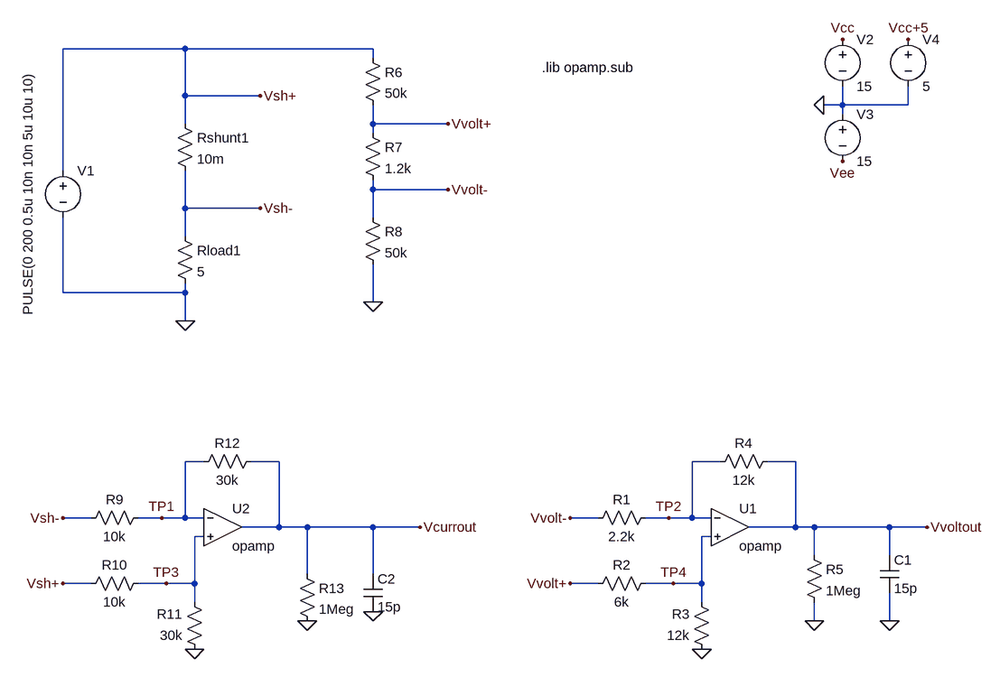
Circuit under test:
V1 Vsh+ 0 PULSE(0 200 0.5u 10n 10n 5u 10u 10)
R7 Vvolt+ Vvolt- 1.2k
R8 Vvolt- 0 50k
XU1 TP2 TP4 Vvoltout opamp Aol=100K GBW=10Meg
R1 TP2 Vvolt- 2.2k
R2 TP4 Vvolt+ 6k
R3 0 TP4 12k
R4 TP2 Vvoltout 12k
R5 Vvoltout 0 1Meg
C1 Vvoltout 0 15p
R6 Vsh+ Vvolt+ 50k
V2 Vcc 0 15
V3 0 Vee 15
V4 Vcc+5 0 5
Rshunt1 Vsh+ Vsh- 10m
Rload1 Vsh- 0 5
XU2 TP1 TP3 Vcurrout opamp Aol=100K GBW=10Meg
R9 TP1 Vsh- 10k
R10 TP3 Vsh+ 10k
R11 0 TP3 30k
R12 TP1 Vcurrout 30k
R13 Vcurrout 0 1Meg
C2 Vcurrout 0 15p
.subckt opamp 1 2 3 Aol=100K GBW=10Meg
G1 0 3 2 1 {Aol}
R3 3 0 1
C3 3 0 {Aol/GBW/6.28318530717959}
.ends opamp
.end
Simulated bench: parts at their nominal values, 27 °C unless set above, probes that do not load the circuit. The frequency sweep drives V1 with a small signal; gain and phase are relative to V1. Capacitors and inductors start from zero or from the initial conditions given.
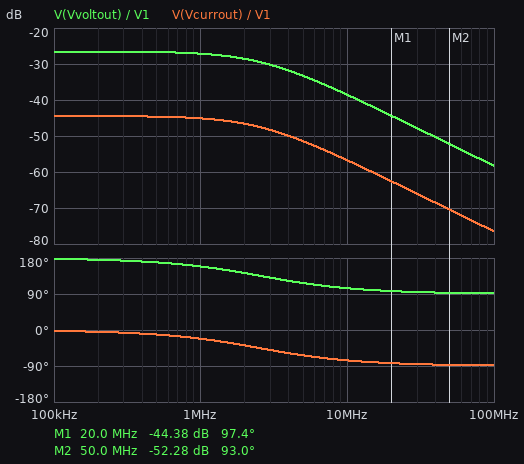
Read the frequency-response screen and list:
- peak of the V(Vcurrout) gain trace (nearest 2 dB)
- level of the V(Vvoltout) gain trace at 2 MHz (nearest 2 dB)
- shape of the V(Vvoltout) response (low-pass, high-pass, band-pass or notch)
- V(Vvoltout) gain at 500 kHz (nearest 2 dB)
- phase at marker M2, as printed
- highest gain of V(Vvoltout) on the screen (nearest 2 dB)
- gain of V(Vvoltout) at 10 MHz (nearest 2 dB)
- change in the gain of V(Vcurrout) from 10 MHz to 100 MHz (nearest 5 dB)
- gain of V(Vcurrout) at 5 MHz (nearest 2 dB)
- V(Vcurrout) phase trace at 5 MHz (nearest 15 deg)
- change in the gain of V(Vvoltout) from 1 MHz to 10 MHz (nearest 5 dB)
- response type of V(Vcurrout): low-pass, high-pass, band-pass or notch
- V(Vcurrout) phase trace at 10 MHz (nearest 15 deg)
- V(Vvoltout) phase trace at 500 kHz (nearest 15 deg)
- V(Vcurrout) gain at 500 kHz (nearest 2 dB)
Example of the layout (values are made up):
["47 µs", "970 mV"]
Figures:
["-44 dB", "-28 dB", "low-pass", "-26 dB", "93.0 deg", "-26 dB", "-38 dB", "-20 dB", "-52 dB", "-60 deg", "-10 dB", "low-pass", "-75 deg", "165 deg", "-44 dB"]
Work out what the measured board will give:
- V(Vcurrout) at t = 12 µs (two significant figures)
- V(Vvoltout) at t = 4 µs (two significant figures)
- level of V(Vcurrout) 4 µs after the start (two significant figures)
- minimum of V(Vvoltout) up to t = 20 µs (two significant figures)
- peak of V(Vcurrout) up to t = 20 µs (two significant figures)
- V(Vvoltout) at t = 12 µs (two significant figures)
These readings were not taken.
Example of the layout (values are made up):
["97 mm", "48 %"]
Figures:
["1.2 V", "-9.4 V", "1.2 V", "-9.4 V", "1.2 V", "-9.4 V"]
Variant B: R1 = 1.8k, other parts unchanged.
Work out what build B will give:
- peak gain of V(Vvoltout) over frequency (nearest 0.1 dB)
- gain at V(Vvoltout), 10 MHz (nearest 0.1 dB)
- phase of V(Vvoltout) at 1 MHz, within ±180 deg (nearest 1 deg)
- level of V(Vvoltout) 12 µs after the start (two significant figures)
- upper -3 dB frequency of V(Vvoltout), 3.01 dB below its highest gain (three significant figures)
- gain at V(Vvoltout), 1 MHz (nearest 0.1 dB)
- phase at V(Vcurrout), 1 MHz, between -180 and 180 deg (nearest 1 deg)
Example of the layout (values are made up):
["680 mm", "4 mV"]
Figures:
["-24.5 dB", "-37.0 dB", "158 deg", "-12 V", "2.46 MHz", "-25.2 dB", "-22 deg"]
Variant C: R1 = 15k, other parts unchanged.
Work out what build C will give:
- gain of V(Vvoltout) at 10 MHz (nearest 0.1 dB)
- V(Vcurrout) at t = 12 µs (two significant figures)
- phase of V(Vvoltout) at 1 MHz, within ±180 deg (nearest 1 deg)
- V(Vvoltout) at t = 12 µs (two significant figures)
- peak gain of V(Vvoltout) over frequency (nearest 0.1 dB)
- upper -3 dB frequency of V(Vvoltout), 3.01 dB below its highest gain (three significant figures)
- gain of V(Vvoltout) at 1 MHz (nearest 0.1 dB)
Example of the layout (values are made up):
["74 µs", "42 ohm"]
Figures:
["-29.2 dB", "1.2 V", "-11 deg", "15 V", "-22.3 dB", "5.07 MHz", "-22.5 dB"]
